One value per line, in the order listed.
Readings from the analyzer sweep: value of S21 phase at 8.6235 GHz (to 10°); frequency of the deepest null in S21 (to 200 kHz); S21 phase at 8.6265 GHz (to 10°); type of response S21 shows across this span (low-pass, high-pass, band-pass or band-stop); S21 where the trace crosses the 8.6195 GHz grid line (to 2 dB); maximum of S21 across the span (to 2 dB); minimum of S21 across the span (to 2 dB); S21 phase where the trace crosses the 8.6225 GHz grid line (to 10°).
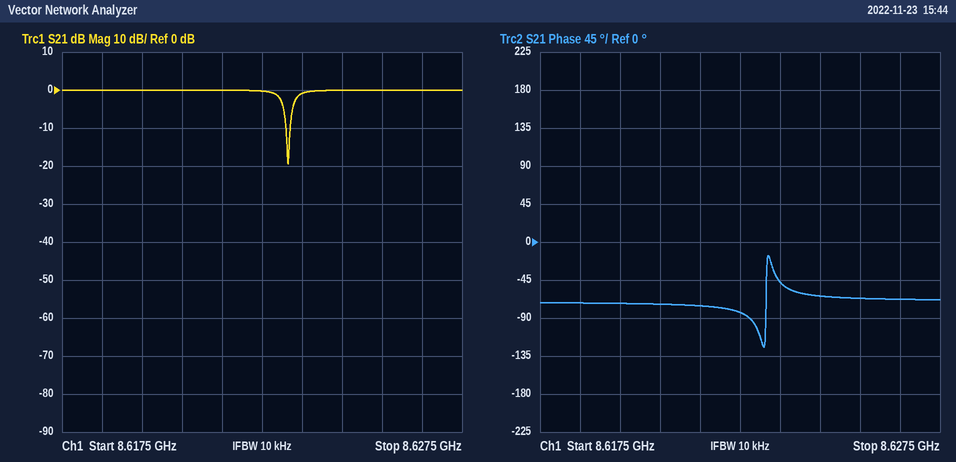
-50°
8.6232 GHz
-70°
band-stop
0 dB
0 dB
-20 dB
-80°
